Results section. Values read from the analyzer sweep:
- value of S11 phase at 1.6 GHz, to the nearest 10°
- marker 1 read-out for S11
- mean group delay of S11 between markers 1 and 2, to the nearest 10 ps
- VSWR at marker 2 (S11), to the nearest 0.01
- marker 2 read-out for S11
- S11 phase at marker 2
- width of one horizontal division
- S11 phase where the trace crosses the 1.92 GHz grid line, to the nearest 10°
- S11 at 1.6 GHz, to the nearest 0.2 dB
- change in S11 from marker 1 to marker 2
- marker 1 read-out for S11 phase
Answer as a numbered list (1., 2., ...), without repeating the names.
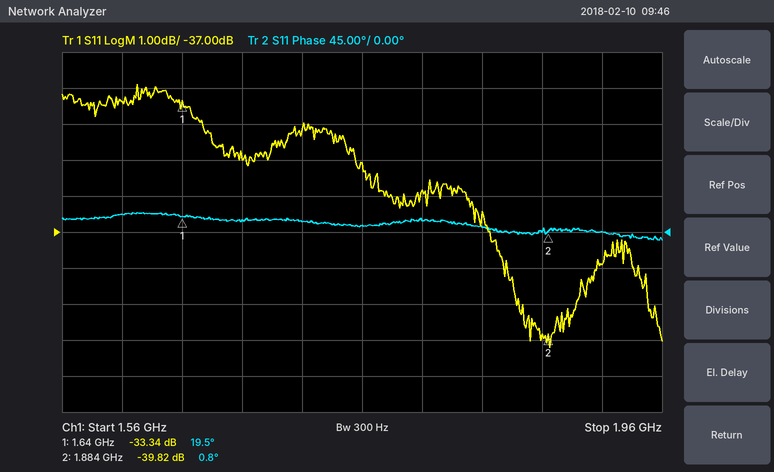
1. 20°
2. -33.34 dB
3. 210 ps
4. 1.02
5. -39.82 dB
6. 0.8°
7. 40 MHz
8. 0°
9. -33.4 dB
10. -6.48 dB
11. 19.5°
